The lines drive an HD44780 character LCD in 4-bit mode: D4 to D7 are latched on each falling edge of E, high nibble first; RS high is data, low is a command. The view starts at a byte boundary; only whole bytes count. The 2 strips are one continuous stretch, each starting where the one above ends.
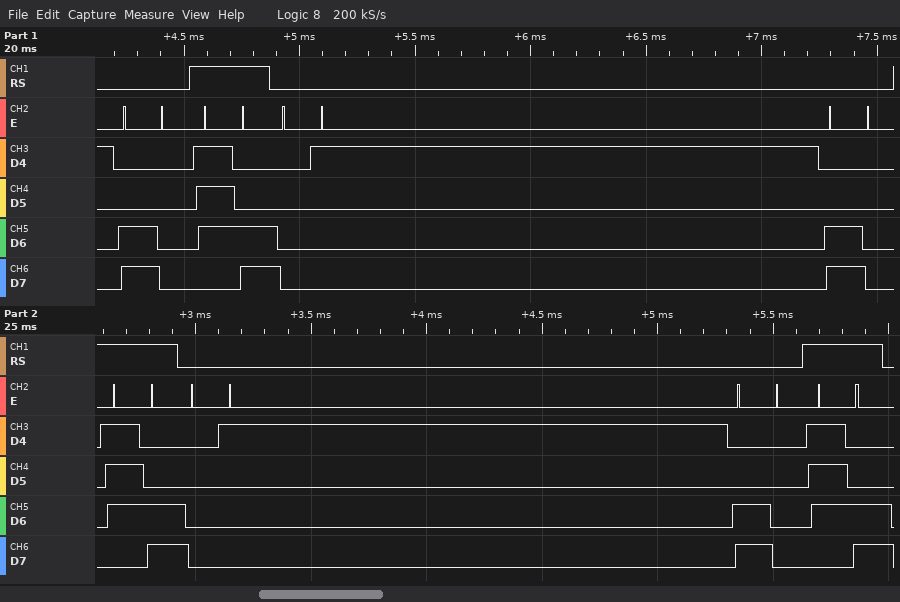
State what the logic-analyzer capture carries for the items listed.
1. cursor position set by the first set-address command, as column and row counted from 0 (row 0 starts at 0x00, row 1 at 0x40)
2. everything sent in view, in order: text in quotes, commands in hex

column 0, row 1
0xC0 "|" 0x01 0xC0 "|" 0x01 0xC0 "|"
